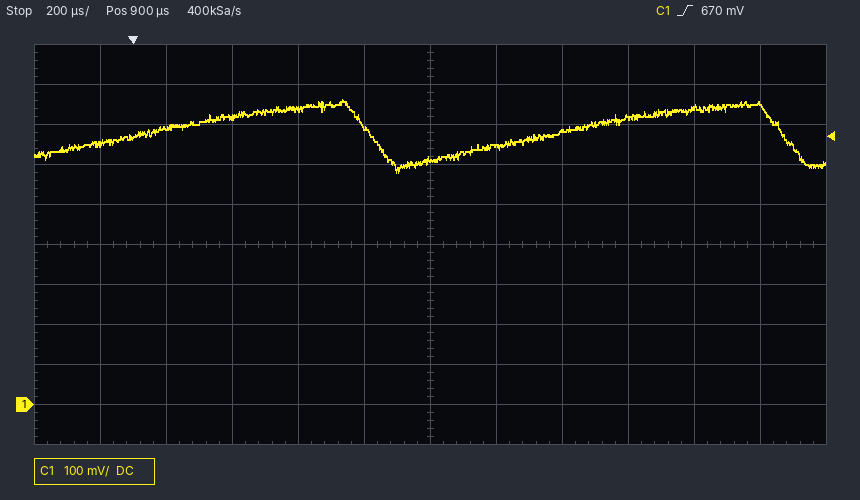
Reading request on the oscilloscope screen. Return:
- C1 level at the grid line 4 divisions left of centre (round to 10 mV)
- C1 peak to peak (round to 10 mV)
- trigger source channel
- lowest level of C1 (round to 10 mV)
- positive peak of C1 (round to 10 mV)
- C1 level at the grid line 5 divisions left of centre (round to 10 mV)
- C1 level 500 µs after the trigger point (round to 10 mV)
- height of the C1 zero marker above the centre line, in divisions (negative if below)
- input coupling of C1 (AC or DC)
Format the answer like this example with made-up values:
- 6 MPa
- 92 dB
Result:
- 690 mV
- 180 mV
- C1
- 580 mV
- 760 mV
- 650 mV
- 740 mV
- -4.0 div
- DC
